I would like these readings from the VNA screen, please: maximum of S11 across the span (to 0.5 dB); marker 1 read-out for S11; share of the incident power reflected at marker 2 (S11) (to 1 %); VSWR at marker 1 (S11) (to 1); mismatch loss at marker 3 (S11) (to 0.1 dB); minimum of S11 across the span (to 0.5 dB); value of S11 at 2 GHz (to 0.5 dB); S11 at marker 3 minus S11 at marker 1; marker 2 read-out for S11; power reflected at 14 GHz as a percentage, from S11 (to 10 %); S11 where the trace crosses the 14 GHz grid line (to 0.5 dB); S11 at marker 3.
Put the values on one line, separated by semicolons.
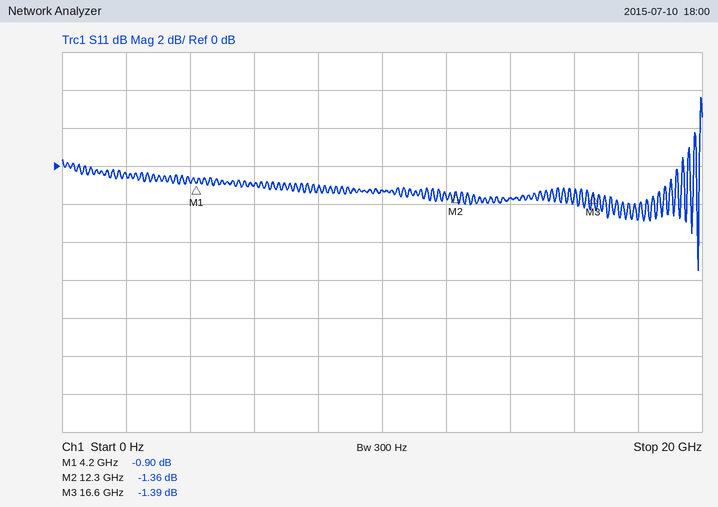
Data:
3.5 dB; -0.90 dB; 73 %; 19; 5.6 dB; -5.5 dB; -0.5 dB; -0.49 dB; -1.36 dB; 70 %; -1.5 dB; -1.39 dB
